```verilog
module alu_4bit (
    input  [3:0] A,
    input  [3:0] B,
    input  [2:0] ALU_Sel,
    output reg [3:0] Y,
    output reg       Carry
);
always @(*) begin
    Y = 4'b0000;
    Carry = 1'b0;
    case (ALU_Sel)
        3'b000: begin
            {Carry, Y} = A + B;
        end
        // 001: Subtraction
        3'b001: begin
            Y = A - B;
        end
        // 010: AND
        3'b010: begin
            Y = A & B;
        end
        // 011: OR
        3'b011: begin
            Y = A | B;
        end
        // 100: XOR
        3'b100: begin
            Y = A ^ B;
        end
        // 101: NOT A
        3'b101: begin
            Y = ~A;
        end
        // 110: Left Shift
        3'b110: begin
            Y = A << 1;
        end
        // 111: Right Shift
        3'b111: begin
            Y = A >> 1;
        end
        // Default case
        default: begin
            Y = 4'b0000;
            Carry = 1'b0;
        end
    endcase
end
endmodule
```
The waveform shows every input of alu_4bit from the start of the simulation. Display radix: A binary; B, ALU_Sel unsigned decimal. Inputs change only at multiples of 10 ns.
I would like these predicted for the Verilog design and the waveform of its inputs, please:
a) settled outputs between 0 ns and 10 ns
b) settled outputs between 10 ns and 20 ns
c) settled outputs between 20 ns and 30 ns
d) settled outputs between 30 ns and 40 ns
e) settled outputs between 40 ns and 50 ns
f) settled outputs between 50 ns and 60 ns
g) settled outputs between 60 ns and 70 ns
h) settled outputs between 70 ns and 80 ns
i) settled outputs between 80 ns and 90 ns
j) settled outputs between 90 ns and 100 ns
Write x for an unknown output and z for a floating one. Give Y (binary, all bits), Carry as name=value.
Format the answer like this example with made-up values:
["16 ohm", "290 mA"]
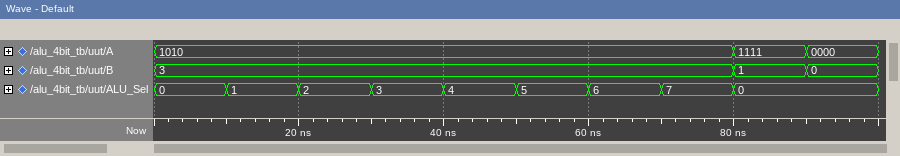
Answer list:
["Y=1101, Carry=0", "Y=0111, Carry=0", "Y=0010, Carry=0", "Y=1011, Carry=0", "Y=1001, Carry=0", "Y=0101, Carry=0", "Y=0100, Carry=0", "Y=0101, Carry=0", "Y=0000, Carry=1", "Y=0000, Carry=0"]
